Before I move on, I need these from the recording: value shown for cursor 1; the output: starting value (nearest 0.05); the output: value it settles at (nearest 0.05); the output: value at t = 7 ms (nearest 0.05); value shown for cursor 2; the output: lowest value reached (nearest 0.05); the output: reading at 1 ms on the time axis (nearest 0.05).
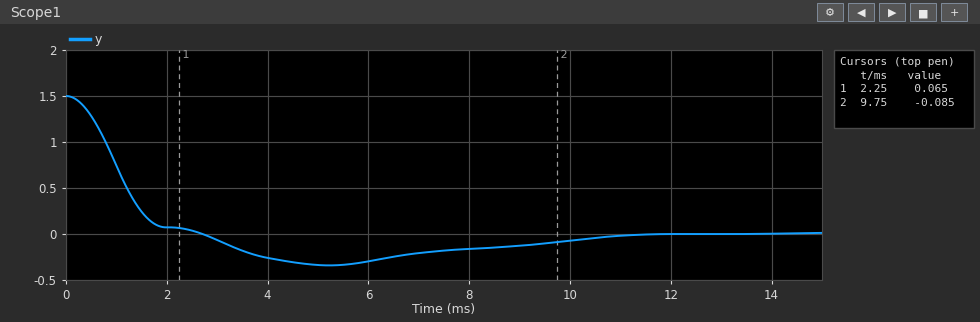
0.065
1.50
0.00
-0.20
-0.085
-0.35
0.75
